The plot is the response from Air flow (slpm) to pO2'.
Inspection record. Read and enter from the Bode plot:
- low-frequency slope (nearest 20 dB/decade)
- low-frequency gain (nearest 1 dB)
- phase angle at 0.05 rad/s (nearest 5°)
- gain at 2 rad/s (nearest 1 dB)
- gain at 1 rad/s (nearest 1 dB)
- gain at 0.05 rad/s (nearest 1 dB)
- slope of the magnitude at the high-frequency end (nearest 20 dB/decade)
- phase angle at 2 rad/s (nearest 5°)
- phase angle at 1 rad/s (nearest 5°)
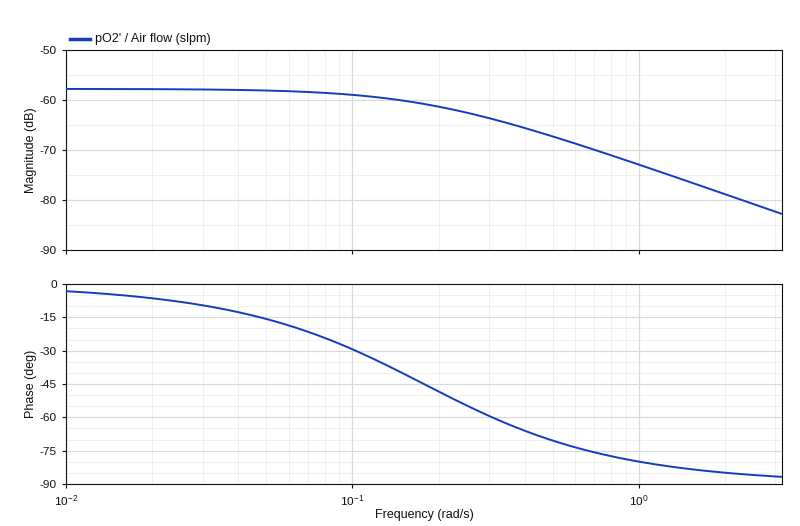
0 dB/decade
-58 dB
-15°
-79 dB
-73 dB
-58 dB
-20 dB/decade
-85°
-80°
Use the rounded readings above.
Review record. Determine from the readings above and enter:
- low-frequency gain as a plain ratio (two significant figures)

0.0013
